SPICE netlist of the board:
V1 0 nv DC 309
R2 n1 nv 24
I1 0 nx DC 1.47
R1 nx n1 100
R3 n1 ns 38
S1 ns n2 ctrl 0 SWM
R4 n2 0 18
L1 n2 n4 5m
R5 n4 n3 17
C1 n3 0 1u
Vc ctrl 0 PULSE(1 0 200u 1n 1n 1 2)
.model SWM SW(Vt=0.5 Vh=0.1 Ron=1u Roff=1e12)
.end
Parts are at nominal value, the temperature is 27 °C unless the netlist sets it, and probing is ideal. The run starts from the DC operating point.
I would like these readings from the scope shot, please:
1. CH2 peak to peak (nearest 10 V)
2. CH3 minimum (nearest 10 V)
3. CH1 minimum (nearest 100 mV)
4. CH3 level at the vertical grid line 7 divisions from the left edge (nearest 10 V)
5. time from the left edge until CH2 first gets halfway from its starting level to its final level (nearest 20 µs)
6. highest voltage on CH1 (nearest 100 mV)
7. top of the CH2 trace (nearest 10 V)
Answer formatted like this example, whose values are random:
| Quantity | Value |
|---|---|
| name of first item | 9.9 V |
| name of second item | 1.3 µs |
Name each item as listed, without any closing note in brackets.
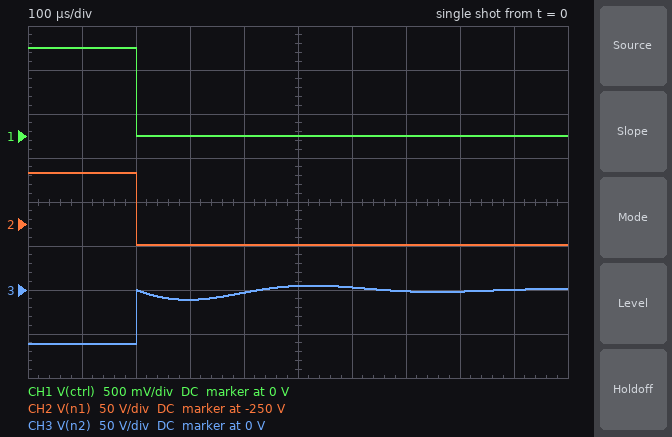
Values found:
| Quantity | Value |
|---|---|
| CH2 peak to peak | 80 V |
| CH3 minimum | -60 V |
| CH1 minimum | 0 V |
| CH3 level at the vertical grid line 7 divisions from the left edge | 0 V |
| time from the left edge until CH2 first gets halfway from its starting level to its final level | 200 µs |
| highest voltage on CH1 | 1.0 V |
| top of the CH2 trace | -190 V |
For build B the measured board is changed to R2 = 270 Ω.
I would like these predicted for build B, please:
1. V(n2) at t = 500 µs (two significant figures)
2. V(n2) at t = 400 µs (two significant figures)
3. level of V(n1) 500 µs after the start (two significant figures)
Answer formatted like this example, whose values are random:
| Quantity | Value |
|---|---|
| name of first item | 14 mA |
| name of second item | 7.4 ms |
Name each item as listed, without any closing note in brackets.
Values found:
| Quantity | Value |
|---|---|
| V(n2) at t = 500 µs | -370 mV |
| V(n2) at t = 400 µs | 250 mV |
| level of V(n1) 500 µs after the start | 88 V |
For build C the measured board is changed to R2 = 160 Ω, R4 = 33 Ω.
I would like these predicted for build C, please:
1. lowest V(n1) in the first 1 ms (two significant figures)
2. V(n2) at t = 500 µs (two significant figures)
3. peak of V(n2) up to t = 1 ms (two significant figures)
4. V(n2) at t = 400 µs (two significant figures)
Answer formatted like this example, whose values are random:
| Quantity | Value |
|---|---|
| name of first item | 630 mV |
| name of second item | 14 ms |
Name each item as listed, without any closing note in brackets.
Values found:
| Quantity | Value |
|---|---|
| lowest V(n1) in the first 1 ms | -74 V |
| V(n2) at t = 500 µs | 860 mV |
| peak of V(n2) up to t = 1 ms | 950 mV |
| V(n2) at t = 400 µs | -920 mV |
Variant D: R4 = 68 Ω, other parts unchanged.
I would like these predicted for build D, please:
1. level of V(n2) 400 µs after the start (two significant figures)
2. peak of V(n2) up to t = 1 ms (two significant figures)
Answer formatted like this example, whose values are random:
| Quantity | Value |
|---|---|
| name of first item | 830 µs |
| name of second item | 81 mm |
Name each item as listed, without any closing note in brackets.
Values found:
| Quantity | Value |
|---|---|
| level of V(n2) 400 µs after the start | -24 V |
| peak of V(n2) up to t = 1 ms | 6.5 V |
